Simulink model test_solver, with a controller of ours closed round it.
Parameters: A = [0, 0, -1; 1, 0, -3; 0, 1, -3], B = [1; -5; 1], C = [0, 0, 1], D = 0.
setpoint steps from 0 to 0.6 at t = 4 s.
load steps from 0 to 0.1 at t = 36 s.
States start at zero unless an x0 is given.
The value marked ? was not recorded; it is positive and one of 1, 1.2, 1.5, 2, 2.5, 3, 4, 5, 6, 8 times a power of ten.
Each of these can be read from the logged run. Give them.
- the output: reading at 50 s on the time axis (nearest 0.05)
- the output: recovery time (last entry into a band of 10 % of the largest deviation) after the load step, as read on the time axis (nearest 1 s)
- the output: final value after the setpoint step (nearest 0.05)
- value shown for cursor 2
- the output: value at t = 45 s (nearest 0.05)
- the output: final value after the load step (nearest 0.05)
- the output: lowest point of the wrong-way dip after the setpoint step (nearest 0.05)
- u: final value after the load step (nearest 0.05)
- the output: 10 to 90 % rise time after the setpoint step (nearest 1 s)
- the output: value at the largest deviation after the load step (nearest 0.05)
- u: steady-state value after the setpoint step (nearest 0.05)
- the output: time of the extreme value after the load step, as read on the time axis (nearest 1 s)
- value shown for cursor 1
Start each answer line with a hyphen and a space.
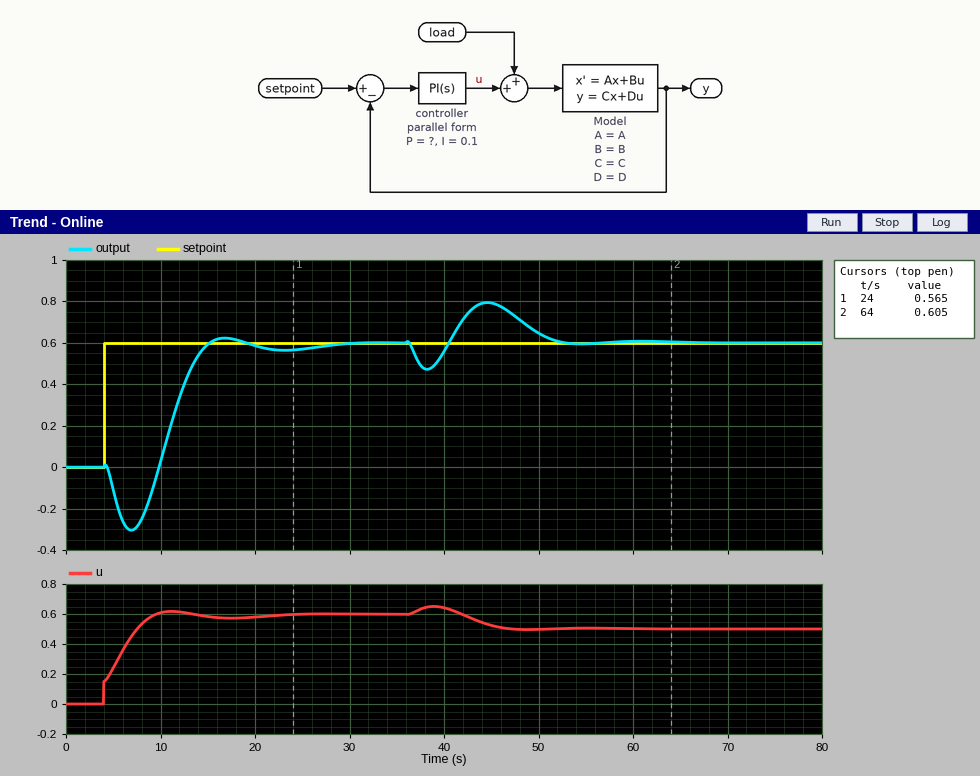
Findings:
- 0.65
- 51 s
- 0.60
- 0.605
- 0.80
- 0.60
- -0.30
- 0.50
- 4 s
- 0.80
- 0.60
- 45 s
- 0.565
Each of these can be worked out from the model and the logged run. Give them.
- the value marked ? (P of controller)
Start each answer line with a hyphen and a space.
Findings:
- 0.25
